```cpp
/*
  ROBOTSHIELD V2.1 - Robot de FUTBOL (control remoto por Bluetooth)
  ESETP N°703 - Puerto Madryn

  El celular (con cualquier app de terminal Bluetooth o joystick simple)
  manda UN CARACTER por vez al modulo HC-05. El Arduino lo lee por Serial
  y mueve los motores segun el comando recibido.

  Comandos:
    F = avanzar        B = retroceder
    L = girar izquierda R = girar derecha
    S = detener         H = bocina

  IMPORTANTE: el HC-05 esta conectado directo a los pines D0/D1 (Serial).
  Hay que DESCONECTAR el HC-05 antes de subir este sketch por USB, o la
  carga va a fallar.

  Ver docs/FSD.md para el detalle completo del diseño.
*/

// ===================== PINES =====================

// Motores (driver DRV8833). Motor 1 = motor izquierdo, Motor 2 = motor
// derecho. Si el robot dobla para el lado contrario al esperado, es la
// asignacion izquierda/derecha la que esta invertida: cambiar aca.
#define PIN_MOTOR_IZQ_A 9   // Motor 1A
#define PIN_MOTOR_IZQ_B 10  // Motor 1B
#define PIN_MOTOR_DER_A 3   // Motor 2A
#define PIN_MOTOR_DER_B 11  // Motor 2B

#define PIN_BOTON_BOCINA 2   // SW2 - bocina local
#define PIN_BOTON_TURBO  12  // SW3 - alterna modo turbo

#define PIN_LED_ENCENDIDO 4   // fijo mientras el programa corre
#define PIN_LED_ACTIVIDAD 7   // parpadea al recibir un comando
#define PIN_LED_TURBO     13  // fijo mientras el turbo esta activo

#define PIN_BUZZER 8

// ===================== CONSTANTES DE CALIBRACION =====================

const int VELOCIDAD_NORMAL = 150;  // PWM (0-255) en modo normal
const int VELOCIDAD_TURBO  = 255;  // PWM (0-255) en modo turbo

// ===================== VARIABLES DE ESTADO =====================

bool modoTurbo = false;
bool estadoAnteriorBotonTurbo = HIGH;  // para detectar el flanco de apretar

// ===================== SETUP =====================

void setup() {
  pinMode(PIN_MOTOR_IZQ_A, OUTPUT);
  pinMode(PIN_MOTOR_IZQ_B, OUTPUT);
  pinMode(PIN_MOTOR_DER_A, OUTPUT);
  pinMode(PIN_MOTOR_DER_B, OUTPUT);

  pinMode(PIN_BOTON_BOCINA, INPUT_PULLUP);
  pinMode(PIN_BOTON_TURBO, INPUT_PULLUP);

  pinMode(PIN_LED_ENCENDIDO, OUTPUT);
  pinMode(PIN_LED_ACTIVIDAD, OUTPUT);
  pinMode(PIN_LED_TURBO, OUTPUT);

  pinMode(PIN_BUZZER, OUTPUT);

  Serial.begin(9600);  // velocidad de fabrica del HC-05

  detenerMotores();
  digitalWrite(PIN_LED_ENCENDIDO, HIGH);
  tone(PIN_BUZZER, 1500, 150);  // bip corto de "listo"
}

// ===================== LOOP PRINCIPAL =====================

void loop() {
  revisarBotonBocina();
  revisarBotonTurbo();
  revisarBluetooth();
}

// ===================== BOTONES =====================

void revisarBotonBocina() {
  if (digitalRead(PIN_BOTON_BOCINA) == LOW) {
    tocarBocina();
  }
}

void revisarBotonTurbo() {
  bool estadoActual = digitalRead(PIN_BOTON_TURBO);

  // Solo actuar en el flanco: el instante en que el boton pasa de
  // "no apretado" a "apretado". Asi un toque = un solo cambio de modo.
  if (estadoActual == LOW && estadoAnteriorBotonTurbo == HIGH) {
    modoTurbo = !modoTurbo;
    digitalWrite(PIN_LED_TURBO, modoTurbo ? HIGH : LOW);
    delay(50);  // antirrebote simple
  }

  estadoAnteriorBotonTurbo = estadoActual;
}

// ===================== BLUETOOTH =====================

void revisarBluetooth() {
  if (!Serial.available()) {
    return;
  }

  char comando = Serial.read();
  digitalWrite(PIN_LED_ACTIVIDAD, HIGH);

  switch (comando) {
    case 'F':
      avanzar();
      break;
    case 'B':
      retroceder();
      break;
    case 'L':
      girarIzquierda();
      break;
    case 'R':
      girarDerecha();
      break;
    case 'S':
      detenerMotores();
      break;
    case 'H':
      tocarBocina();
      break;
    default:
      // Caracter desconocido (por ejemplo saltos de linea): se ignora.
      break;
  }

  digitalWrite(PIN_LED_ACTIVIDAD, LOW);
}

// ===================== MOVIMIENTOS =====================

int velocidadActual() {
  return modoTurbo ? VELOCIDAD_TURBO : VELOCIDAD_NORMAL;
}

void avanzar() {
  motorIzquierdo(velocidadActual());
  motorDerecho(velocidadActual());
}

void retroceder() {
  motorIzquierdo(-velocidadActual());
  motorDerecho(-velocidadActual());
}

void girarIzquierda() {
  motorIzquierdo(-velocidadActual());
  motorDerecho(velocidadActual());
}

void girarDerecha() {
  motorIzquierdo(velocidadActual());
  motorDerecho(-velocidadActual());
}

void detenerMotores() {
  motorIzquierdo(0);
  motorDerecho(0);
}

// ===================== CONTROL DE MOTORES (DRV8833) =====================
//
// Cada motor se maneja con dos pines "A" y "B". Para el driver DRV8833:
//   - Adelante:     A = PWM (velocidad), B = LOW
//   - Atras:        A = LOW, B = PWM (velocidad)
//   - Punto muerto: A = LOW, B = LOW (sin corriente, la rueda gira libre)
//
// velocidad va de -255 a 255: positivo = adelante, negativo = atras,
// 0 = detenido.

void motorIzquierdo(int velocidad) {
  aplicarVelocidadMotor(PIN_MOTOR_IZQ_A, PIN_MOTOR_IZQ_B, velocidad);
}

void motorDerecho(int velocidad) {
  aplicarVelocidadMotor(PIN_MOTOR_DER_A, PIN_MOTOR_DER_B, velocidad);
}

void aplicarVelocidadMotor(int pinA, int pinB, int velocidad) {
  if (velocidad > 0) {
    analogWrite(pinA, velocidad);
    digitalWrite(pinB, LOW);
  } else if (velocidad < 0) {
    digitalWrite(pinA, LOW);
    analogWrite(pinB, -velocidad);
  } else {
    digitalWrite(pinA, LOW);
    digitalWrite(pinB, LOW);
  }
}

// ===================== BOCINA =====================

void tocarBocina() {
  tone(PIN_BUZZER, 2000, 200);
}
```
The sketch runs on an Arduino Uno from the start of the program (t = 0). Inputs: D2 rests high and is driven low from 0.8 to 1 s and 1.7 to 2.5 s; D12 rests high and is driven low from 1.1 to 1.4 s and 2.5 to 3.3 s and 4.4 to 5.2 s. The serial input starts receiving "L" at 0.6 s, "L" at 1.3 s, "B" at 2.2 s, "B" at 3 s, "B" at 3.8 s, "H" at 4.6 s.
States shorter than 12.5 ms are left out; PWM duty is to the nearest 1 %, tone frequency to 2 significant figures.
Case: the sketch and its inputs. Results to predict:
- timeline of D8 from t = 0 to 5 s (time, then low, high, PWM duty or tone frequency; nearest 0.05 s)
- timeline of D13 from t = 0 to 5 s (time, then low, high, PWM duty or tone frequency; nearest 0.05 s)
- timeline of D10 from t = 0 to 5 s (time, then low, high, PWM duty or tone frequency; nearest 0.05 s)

0 s tone 1500 Hz; 0.15 s low; 0.8 s tone 2000 Hz; 1.2 s low; 1.7 s tone 2000 Hz; 2.7 s low; 4.6 s tone 2000 Hz; 4.8 s low
0 s low; 1.1 s high; 2.5 s low; 4.4 s high
0 s low; 0.6 s PWM 59 %; 1.3 s high; 3 s PWM 59 %
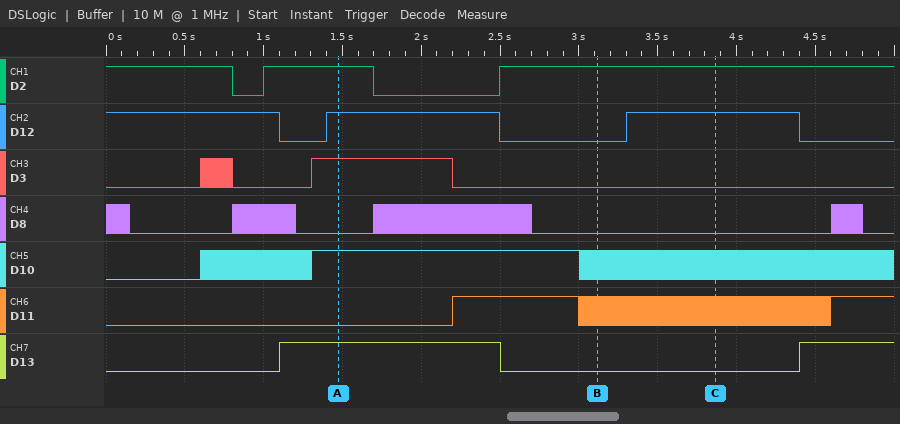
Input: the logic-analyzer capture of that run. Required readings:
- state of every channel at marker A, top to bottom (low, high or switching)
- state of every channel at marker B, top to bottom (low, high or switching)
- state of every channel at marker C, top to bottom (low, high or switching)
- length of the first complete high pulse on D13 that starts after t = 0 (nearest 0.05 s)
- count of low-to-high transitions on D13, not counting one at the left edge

D2 high, D12 high, D3 high, D8 low, D10 high, D11 low, D13 high
D2 high, D12 low, D3 low, D8 low, D10 switching, D11 switching, D13 low
D2 high, D12 high, D3 low, D8 low, D10 switching, D11 switching, D13 low
1.40 s
2
